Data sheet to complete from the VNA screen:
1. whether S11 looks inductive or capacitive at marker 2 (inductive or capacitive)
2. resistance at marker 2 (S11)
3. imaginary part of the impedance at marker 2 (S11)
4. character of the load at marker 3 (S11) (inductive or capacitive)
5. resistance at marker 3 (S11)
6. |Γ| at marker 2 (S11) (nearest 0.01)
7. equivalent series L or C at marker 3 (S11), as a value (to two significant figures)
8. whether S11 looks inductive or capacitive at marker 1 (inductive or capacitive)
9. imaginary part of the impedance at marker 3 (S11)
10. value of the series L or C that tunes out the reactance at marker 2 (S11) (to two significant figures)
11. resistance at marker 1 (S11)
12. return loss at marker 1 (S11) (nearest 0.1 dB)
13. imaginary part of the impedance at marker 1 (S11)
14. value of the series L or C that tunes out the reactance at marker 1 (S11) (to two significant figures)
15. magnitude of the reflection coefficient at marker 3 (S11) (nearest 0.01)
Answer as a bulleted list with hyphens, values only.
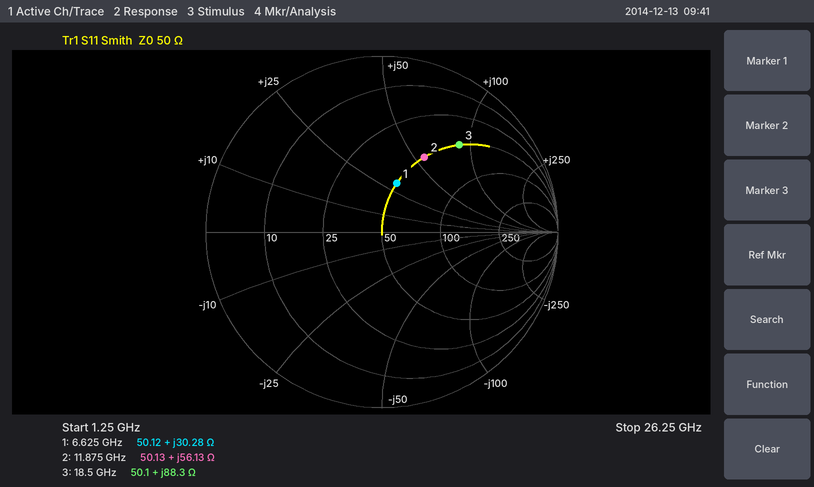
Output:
- inductive
- 50.13 Ω
- +56.13 Ω
- inductive
- 50.1 Ω
- 0.49
- 760 pH
- inductive
- +88.3 Ω
- 240 fF
- 50.12 Ω
- 10.8 dB
- +30.28 Ω
- 790 fF
- 0.66
